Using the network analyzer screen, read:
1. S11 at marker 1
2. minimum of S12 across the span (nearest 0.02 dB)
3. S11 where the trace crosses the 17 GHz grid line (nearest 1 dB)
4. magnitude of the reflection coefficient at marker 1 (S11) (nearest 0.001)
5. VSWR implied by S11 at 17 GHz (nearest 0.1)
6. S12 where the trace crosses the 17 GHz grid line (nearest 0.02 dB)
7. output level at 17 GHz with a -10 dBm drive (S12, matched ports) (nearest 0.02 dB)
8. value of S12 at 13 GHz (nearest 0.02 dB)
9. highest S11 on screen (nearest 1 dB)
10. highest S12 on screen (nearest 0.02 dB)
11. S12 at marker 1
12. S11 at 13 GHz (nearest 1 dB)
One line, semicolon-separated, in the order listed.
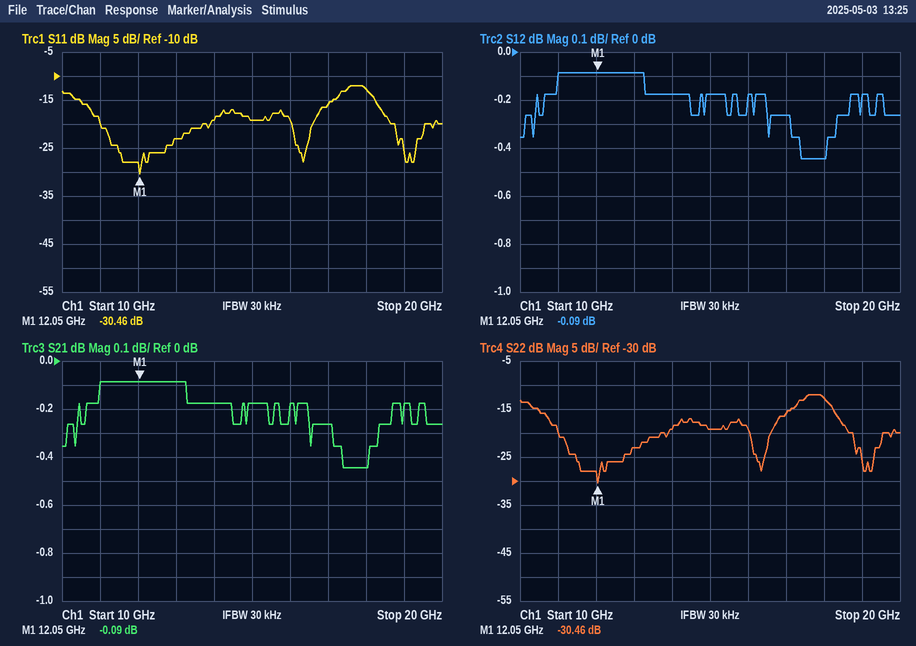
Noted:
-30.46 dB; -0.44 dB; -16 dB; 0.030; 1.4; -0.26 dB; -10.26 dBm; -0.08 dB; -12 dB; -0.08 dB; -0.09 dB; -23 dB
